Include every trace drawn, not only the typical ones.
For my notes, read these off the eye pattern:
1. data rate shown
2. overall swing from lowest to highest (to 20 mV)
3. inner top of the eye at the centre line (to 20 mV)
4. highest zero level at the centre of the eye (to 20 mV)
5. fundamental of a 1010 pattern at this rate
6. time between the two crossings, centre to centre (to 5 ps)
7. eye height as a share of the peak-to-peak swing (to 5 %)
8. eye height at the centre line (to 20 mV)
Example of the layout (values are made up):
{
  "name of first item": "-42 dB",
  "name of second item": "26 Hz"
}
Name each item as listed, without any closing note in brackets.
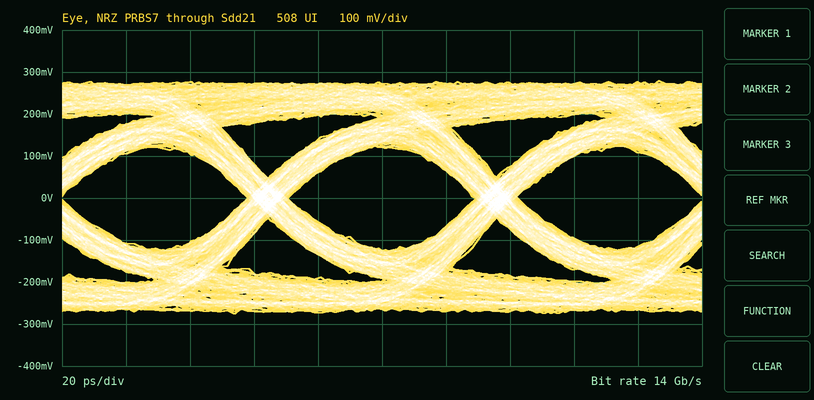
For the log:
{
  "data rate shown": "14 Gb/s",
  "overall swing from lowest to highest": "560 mV",
  "inner top of the eye at the centre line": "120 mV",
  "highest zero level at the centre of the eye": "-120 mV",
  "fundamental of a 1010 pattern at this rate": "7 GHz",
  "time between the two crossings, centre to centre": "70 ps",
  "eye height as a share of the peak-to-peak swing": "45 %",
  "eye height at the centre line": "240 mV"
}
